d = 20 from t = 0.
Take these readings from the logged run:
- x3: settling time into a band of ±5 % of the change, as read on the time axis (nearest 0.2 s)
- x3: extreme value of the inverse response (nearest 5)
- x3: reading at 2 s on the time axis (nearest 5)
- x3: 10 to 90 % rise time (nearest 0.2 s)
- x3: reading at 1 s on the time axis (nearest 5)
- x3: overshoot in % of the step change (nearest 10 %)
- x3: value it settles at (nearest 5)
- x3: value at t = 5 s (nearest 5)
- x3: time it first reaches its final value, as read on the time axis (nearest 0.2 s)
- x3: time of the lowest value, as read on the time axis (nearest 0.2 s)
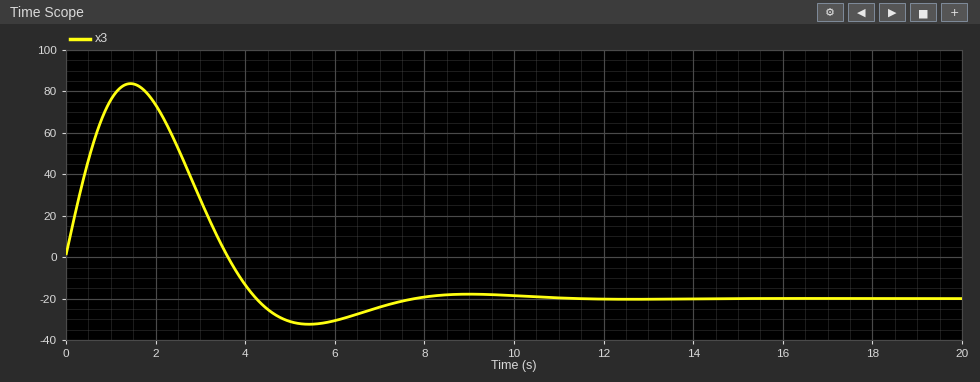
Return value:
10.4 s
85
75
0.6 s
75
60 %
-20
-30
4.2 s
5.4 s
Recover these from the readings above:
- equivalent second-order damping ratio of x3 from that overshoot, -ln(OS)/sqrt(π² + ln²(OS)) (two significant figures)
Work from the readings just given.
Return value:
0.16
